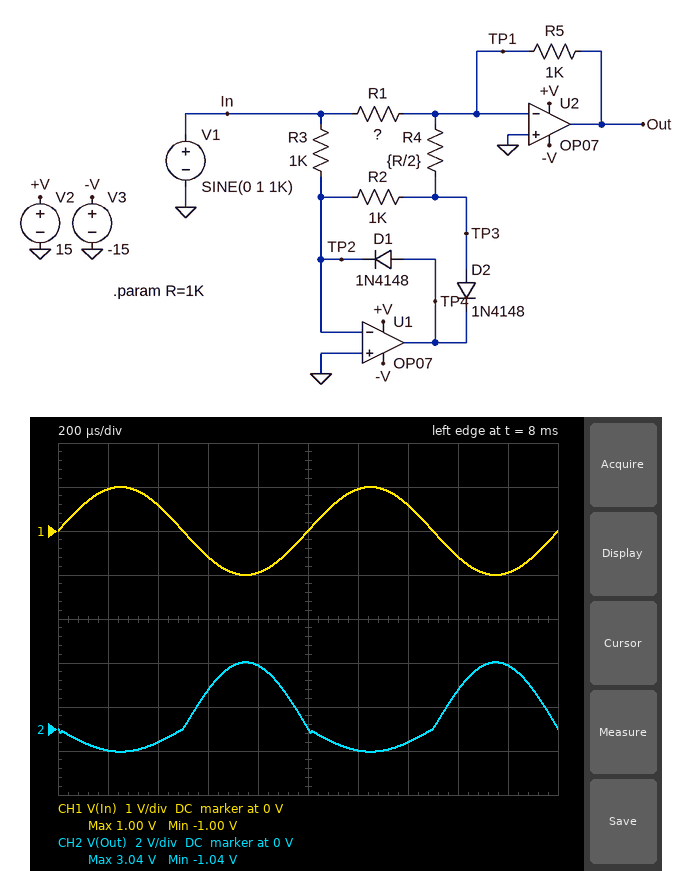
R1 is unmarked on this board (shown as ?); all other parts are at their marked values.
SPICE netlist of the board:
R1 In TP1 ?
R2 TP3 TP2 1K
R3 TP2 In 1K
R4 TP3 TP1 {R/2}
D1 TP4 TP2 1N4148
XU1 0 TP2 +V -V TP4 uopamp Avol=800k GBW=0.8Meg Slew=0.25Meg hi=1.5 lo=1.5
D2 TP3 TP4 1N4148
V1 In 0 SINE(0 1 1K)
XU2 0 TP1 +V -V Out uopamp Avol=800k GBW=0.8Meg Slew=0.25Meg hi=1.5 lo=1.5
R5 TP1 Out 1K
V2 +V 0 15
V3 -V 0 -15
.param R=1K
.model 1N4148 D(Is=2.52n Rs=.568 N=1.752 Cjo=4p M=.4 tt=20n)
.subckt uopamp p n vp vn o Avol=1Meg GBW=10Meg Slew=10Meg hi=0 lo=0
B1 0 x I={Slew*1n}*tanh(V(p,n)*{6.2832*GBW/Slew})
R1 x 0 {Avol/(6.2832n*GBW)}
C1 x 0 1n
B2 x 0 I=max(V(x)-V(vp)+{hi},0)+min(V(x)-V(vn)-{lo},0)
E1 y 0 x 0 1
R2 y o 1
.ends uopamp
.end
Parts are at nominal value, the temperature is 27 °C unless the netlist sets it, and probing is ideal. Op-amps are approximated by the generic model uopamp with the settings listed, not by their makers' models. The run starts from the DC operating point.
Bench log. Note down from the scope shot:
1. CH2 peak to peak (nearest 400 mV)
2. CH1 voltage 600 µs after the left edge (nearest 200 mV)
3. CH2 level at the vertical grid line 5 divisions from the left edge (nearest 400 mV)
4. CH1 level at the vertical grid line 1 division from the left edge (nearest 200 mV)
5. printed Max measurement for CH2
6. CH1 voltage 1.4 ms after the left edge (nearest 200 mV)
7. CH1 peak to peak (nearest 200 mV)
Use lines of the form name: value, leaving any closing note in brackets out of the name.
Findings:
CH2 peak to peak: 4.0 V
CH1 voltage 600 µs after the left edge: -600 mV
CH2 level at the vertical grid line 5 divisions from the left edge: 0 V
CH1 level at the vertical grid line 1 division from the left edge: 1.0 V
printed Max measurement for CH2: 3.04 V
CH1 voltage 1.4 ms after the left edge: 600 mV
CH1 peak to peak: 2.0 V
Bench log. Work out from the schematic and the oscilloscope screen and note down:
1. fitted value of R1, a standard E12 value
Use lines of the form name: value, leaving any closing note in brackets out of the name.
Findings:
fitted value of R1, a standard E12 value: 330 Ω
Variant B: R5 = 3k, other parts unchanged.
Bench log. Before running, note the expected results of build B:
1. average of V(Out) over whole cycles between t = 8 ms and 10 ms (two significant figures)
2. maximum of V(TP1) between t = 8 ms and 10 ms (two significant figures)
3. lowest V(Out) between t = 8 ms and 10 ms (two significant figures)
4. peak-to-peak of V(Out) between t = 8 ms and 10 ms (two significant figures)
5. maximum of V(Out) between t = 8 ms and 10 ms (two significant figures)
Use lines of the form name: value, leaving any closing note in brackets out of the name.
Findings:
average of V(Out) over whole cycles between t = 8 ms and 10 ms: 1.9 V
maximum of V(TP1) between t = 8 ms and 10 ms: 13 mV
lowest V(Out) between t = 8 ms and 10 ms: -3.1 V
peak-to-peak of V(Out) between t = 8 ms and 10 ms: 12 V
maximum of V(Out) between t = 8 ms and 10 ms: 9.1 V
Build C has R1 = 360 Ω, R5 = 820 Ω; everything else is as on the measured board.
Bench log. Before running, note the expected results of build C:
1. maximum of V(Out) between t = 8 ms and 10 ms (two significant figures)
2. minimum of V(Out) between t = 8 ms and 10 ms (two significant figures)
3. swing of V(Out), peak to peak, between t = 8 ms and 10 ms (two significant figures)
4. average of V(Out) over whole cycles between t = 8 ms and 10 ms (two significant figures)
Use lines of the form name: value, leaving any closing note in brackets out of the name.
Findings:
maximum of V(Out) between t = 8 ms and 10 ms: 2.3 V
minimum of V(Out) between t = 8 ms and 10 ms: -640 mV
swing of V(Out), peak to peak, between t = 8 ms and 10 ms: 2.9 V
average of V(Out) over whole cycles between t = 8 ms and 10 ms: 520 mV
